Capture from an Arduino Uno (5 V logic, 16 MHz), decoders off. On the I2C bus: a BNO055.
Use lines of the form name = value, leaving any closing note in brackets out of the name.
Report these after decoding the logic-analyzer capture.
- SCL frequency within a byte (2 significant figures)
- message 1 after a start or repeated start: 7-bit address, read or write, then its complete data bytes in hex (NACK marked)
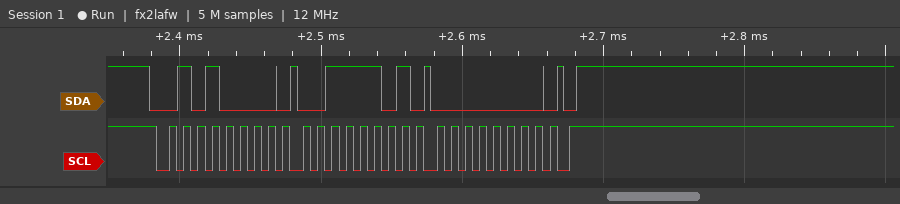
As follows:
SCL frequency within a byte = 100 kHz
message 1 after a start or repeated start: 7-bit address, read or write, then its complete data bytes in hex = 0x28 write: 3D 00
